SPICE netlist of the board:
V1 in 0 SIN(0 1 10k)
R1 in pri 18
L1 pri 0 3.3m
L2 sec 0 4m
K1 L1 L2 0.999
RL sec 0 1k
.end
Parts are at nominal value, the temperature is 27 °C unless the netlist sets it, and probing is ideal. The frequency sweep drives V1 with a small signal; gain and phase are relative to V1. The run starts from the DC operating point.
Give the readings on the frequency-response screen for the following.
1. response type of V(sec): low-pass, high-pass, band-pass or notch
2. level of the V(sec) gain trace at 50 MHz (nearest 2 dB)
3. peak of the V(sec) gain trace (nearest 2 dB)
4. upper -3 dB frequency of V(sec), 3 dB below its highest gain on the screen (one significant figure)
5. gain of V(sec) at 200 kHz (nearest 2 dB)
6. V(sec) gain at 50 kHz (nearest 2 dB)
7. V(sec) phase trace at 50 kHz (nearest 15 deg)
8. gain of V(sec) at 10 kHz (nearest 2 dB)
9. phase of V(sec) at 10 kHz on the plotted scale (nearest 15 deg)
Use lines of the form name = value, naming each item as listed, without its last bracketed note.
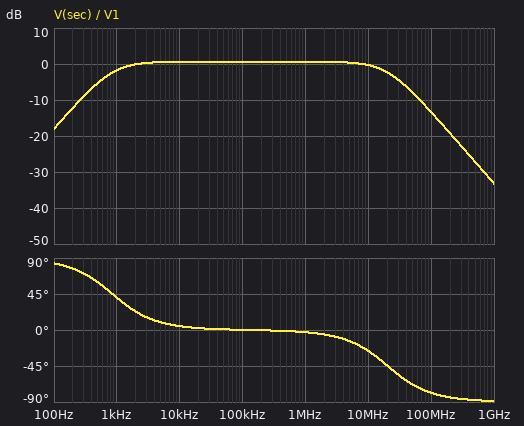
response type of V(sec): low-pass, high-pass, band-pass or notch = band-pass
level of the V(sec) gain trace at 50 MHz = -8 dB
peak of the V(sec) gain trace = 0 dB
upper -3 dB frequency of V(sec), 3 dB below its highest gain on the screen = 20 MHz
gain of V(sec) at 200 kHz = 0 dB
V(sec) gain at 50 kHz = 0 dB
V(sec) phase trace at 50 kHz = 0 deg
gain of V(sec) at 10 kHz = 0 dB
phase of V(sec) at 10 kHz on the plotted scale = 0 deg
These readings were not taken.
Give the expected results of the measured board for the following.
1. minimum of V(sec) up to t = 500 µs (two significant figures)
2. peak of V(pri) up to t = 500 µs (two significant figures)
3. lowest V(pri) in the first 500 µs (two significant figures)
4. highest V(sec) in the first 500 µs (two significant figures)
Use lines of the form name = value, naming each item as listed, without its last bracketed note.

minimum of V(sec) up to t = 500 µs = -1.1 V
peak of V(pri) up to t = 500 µs = 970 mV
lowest V(pri) in the first 500 µs = -1.0 V
highest V(sec) in the first 500 µs = 1.1 V
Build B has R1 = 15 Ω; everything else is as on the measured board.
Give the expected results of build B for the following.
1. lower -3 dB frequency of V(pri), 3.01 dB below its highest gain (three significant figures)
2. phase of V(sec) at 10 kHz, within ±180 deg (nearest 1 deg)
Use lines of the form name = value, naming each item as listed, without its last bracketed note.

lower -3 dB frequency of V(pri), 3.01 dB below its highest gain = 737 Hz
phase of V(sec) at 10 kHz, within ±180 deg = 4 deg
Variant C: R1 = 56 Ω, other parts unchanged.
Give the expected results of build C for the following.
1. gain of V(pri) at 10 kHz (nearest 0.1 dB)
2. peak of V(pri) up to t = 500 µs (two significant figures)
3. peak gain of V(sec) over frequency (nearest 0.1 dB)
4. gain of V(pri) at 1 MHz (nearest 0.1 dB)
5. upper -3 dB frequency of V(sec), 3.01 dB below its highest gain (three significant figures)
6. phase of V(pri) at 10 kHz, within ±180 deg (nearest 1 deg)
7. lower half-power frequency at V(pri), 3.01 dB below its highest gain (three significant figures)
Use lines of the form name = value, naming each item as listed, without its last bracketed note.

gain of V(pri) at 10 kHz = -0.8 dB
peak of V(pri) up to t = 500 µs = 910 mV
peak gain of V(sec) over frequency = 0.3 dB
gain of V(pri) at 1 MHz = -0.6 dB
upper -3 dB frequency of V(sec), 3.01 dB below its highest gain = 21.3 MHz
phase of V(pri) at 10 kHz, within ±180 deg = 14 deg
lower half-power frequency at V(pri), 3.01 dB below its highest gain = 2.91 kHz
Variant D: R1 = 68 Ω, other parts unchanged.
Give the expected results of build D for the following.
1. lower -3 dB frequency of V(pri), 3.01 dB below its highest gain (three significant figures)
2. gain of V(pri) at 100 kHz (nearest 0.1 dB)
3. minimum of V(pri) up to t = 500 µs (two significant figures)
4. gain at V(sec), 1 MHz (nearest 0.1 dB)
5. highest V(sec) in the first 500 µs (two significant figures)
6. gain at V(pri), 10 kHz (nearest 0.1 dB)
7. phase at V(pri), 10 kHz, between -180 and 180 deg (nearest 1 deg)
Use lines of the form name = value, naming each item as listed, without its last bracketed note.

lower -3 dB frequency of V(pri), 3.01 dB below its highest gain = 3.60 kHz
gain of V(pri) at 100 kHz = -0.7 dB
minimum of V(pri) up to t = 500 µs = -950 mV
gain at V(sec), 1 MHz = 0.1 dB
highest V(sec) in the first 500 µs = 970 mV
gain at V(pri), 10 kHz = -1.1 dB
phase at V(pri), 10 kHz, between -180 and 180 deg = 17 deg
